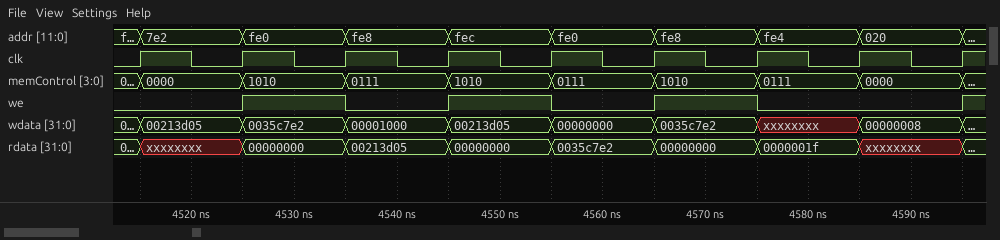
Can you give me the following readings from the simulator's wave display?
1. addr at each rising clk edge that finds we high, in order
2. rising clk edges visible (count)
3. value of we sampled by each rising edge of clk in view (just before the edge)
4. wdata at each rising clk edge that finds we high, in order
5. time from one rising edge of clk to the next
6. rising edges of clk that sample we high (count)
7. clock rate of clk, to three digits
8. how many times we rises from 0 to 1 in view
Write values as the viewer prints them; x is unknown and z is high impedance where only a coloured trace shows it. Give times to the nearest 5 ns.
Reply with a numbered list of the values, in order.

1. fe0, fec, fe8
2. 9
3. 0 0 1 0 1 0 1 0 0
4. 0035c7e2, 00213d05, 0035c7e2
5. 10 ns
6. 3
7. 100 MHz
8. 4
